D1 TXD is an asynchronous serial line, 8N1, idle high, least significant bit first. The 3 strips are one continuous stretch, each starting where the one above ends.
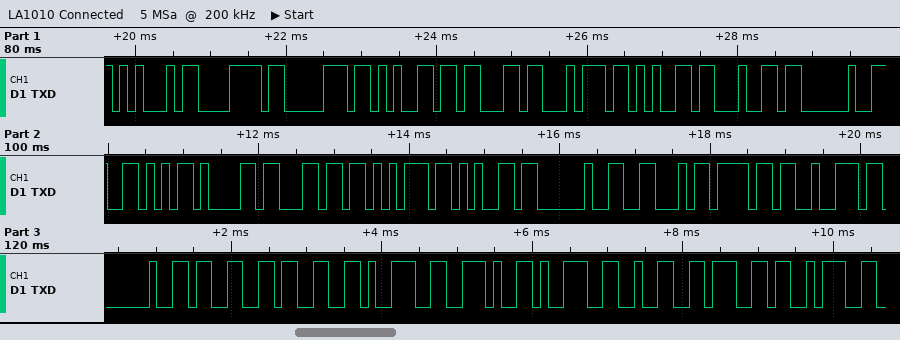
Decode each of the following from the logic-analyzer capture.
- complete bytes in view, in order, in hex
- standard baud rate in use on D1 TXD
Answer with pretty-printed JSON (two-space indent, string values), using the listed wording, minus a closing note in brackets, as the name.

{
  "complete bytes in view, in order, in hex": "45 78 70 65 63 74 65 64 20 56 61 6C 75 65 20 46 6F 72 20 33 33 39 2E 39 32 67 3A",
  "standard baud rate in use on D1 TXD": "9600 baud"
}
